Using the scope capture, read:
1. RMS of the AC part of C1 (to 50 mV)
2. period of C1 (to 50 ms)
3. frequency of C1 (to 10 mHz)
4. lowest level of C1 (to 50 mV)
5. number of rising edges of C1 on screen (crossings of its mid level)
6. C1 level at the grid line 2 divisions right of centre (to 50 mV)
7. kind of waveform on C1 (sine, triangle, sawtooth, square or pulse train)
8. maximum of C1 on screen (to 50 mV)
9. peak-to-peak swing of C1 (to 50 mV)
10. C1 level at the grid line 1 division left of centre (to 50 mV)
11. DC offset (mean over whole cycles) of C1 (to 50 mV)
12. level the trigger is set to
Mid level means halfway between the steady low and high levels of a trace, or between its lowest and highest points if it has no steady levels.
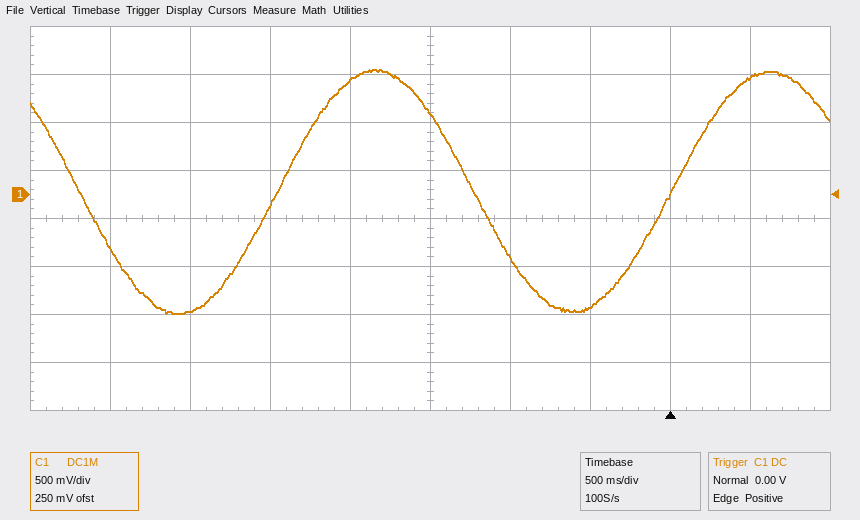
900 mV
2.45 s
410 mHz
-1.25 V
2
-1.15 V
sine
1.30 V
2.55 V
1.20 V
50 mV
0.00 V
